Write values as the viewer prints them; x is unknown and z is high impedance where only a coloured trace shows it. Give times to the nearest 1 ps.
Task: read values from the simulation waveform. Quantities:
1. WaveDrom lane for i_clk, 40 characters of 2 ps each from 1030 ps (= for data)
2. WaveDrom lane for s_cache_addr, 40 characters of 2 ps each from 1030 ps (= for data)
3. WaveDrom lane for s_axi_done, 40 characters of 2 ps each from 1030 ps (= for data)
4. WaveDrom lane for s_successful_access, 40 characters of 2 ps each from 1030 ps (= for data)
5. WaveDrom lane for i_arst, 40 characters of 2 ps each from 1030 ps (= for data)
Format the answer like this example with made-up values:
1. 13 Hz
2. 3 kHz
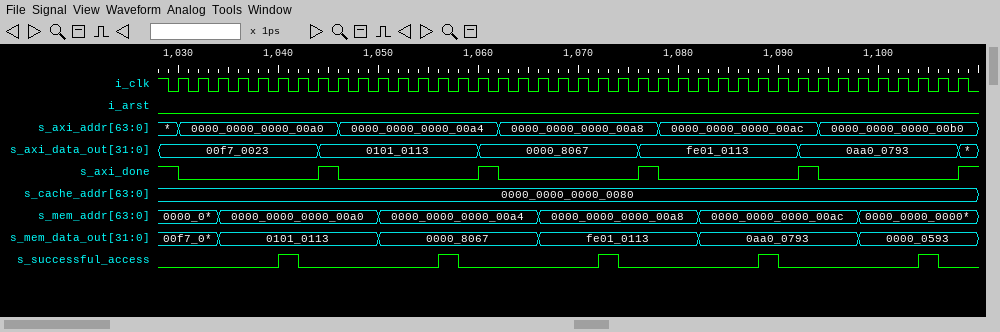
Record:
1. {name: 'i_clk', wave: 'p.......................................'}
2. {name: 's_cache_addr', wave: '=.......................................', data: '0000_0000_0000_0080'}
3. {name: 's_axi_done', wave: '0......10......10......10......10......1'}
4. {name: 's_successful_access', wave: '0....10......10......10......10......10.'}
5. {name: 'i_arst', wave: '0.......................................'}
